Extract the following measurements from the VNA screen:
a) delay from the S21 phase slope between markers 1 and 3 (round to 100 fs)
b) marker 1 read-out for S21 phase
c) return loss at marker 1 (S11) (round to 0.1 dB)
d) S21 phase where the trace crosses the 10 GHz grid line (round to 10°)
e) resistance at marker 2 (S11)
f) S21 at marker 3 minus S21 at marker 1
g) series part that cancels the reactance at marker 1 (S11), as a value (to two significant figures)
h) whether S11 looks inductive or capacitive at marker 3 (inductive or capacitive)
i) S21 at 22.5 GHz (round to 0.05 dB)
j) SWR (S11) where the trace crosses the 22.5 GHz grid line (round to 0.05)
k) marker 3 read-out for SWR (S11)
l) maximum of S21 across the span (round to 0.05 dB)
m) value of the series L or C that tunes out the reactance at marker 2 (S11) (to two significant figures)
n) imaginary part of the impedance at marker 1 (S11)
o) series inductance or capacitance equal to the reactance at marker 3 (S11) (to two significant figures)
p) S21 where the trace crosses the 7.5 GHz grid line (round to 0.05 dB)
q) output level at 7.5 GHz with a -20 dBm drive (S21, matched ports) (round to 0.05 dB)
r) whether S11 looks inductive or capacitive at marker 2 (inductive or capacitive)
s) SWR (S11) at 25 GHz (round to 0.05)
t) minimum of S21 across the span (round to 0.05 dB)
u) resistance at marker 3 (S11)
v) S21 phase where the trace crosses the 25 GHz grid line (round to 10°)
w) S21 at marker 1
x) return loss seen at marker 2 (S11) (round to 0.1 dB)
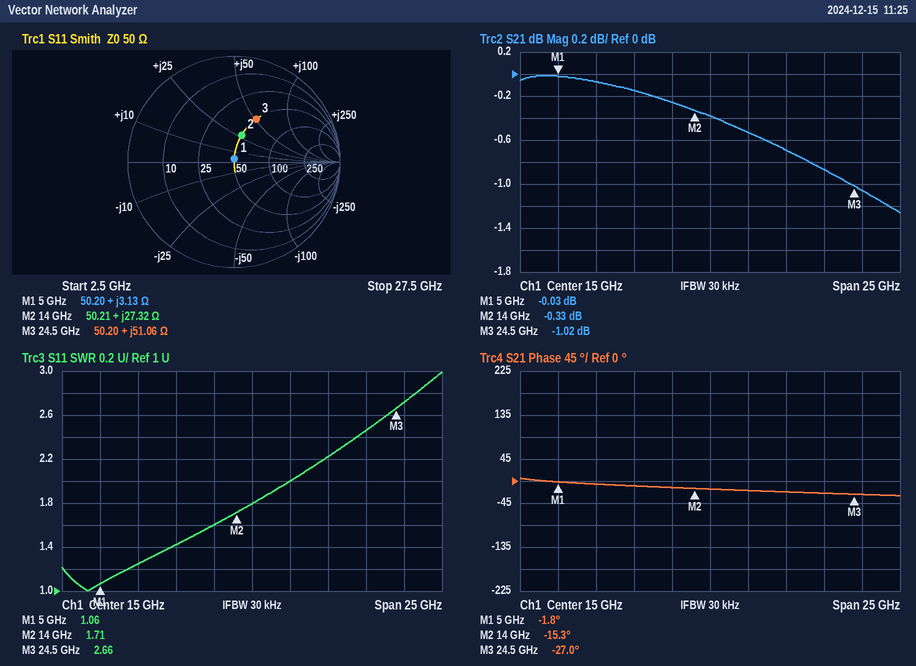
3.6 ps
-1.8°
30.1 dB
-10°
50.21 Ω
-0.99 dB
10 pF
inductive
-0.85 dB
2.45
2.66
0.00 dB
420 fF
+3.13 Ω
330 pH
-0.05 dB
-20.05 dBm
inductive
2.70
-1.25 dB
50.20 Ω
-30°
-0.03 dB
11.6 dB
